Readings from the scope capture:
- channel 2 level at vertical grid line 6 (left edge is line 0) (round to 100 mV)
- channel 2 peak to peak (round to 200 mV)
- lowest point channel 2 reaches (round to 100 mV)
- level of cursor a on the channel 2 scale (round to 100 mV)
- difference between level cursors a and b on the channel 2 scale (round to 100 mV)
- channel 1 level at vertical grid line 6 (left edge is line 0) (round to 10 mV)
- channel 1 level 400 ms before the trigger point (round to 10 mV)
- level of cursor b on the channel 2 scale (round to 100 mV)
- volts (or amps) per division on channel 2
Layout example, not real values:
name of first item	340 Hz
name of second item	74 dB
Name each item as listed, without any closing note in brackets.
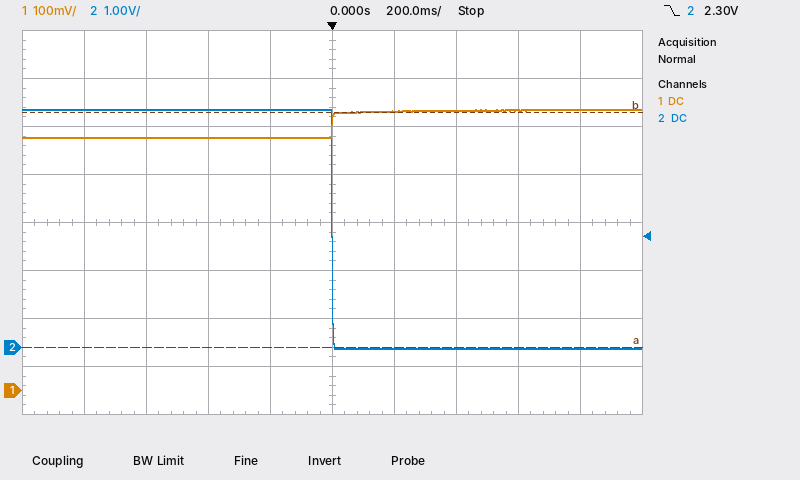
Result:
channel 2 level at vertical grid line 6 (left edge is line 0)	0.0 V
channel 2 peak to peak	5.0 V
lowest point channel 2 reaches	0.0 V
level of cursor a on the channel 2 scale	0.0 V
difference between level cursors a and b on the channel 2 scale	4.9 V
channel 1 level at vertical grid line 6 (left edge is line 0)	580 mV
channel 1 level 400 ms before the trigger point	530 mV
level of cursor b on the channel 2 scale	4.9 V
volts (or amps) per division on channel 2	1 V
